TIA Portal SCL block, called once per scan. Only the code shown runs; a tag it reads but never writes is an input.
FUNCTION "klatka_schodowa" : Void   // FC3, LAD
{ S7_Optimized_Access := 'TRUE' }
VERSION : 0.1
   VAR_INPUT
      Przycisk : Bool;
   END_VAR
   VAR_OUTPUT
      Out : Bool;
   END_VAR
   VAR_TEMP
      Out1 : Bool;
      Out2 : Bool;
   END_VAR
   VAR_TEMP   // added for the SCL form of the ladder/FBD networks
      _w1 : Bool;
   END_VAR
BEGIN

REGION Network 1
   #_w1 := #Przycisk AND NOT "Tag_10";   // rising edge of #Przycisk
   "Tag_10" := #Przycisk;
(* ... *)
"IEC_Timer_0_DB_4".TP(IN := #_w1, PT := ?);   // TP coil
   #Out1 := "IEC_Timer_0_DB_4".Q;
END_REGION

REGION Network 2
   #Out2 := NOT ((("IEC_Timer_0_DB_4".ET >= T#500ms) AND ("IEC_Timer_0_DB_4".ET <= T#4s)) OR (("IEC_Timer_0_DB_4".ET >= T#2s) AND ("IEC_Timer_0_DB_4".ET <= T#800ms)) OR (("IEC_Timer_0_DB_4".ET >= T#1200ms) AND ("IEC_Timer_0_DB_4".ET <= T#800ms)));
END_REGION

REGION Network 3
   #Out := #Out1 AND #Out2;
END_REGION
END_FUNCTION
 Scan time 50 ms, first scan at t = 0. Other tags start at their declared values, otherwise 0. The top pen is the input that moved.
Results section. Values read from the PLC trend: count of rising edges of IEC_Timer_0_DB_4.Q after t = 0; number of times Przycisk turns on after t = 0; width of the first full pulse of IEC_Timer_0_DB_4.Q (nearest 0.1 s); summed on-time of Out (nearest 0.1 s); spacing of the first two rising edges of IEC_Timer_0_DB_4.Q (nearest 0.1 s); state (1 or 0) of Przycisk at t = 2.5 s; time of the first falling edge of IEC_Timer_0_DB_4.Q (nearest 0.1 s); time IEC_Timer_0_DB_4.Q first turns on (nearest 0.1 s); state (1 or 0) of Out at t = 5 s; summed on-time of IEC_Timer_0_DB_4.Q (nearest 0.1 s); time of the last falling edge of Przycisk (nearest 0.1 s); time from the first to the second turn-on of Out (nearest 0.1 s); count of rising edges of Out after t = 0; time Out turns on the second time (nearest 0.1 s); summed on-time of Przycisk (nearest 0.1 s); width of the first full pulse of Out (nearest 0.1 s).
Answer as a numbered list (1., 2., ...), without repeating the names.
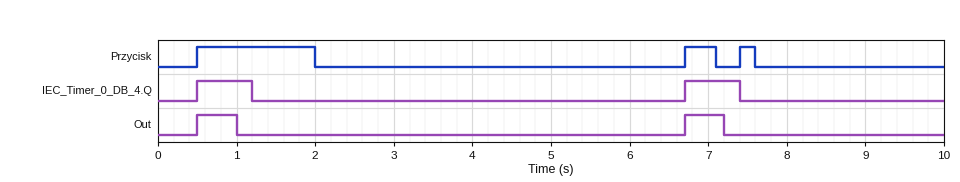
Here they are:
1. 2
2. 3
3. 0.7 s
4. 1.0 s
5. 6.2 s
6. 0
7. 1.2 s
8. 0.5 s
9. 0
10. 1.4 s
11. 7.6 s
12. 6.2 s
13. 2
14. 6.7 s
15. 2.1 s
16. 0.5 s
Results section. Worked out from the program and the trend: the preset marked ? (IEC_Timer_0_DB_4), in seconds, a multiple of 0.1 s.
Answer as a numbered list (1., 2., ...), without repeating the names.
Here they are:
1. 0.7 s
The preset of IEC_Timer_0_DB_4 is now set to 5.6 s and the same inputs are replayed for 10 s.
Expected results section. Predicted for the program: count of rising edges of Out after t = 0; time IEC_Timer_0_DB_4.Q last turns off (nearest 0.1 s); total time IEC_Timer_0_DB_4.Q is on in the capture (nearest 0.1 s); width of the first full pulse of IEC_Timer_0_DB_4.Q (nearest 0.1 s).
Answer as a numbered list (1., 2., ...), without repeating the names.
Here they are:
1. 3
2. 6.1 s
3. 8.9 s
4. 5.6 s
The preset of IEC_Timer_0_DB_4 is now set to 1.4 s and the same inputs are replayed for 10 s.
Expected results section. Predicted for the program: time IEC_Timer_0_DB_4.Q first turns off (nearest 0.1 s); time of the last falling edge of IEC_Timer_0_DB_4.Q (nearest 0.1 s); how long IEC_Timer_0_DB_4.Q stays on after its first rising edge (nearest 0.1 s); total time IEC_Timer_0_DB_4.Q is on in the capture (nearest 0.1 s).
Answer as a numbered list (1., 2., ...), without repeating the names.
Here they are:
1. 1.9 s
2. 8.1 s
3. 1.4 s
4. 2.8 s
